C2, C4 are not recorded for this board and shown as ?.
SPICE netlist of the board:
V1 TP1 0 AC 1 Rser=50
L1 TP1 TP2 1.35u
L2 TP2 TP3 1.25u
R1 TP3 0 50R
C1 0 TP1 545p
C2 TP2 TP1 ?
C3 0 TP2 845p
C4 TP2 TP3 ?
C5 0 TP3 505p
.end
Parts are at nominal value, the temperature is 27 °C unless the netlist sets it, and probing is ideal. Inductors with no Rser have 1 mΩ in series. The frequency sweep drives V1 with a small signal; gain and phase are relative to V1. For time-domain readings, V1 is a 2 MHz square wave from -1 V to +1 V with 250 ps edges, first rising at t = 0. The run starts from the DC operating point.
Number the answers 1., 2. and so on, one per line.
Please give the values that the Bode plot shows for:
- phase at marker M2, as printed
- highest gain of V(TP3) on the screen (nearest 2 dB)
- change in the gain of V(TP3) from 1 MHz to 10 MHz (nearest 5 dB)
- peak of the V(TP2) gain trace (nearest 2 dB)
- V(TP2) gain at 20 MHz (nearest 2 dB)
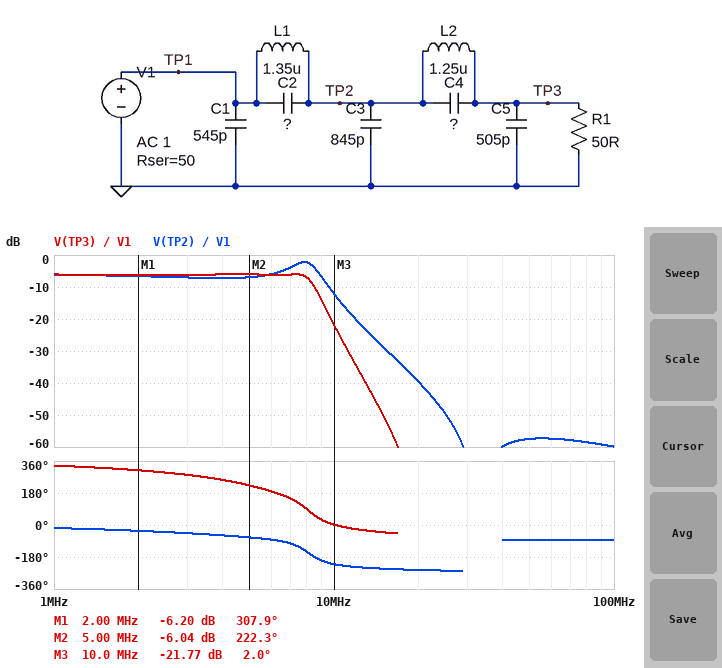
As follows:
1. 222.3 deg
2. -6 dB
3. -15 dB
4. -2 dB
5. -40 dB
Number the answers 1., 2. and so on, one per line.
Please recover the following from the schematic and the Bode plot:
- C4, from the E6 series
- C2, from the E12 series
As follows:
1. 47 pF
2. 18 pF
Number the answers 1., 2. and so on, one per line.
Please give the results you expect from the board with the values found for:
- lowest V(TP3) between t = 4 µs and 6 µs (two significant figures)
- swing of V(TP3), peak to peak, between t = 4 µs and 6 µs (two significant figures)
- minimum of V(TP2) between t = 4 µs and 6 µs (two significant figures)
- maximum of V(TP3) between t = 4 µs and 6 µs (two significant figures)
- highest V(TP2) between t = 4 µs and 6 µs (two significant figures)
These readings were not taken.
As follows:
1. -640 mV
2. 1.3 V
3. -580 mV
4. 640 mV
5. 580 mV
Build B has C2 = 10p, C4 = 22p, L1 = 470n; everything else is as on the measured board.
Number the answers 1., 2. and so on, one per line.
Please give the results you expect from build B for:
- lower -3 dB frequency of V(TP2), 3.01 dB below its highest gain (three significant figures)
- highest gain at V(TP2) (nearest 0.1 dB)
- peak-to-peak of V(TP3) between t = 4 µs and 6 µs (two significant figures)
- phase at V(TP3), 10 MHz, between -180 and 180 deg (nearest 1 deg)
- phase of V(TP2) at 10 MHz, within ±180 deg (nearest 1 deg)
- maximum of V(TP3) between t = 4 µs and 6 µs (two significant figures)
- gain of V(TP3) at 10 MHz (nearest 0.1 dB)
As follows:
1. 10.1 MHz
2. -1.8 dB
3. 1.1 V
4. 129 deg
5. -95 deg
6. 540 mV
7. -12.9 dB
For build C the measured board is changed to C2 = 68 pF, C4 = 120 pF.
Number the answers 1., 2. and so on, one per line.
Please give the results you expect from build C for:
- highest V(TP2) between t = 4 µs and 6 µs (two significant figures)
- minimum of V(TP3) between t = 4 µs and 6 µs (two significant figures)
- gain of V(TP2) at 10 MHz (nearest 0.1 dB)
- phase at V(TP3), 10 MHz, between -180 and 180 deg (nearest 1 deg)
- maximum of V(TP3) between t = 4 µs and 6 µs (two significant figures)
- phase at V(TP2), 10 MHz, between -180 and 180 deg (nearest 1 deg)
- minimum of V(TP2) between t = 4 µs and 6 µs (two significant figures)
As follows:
1. 600 mV
2. -660 mV
3. -18.6 dB
4. -14 deg
5. 660 mV
6. 129 deg
7. -600 mV
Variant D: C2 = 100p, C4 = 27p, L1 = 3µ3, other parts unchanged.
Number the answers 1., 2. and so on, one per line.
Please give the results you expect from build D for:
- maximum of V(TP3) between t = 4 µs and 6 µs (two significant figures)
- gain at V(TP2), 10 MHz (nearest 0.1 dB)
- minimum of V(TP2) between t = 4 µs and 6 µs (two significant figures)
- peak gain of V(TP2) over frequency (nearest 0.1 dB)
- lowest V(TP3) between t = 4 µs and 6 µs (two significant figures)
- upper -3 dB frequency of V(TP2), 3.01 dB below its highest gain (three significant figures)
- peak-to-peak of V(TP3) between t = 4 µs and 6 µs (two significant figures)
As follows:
1. 590 mV
2. -35.1 dB
3. -530 mV
4. -6.0 dB
5. -590 mV
6. 3.56 MHz
7. 1.2 V
